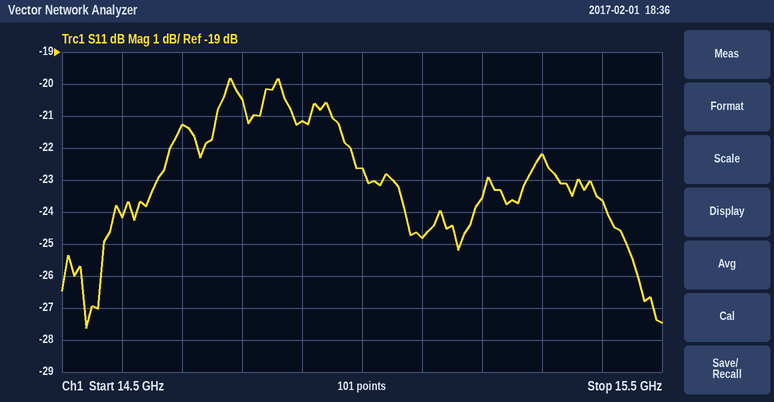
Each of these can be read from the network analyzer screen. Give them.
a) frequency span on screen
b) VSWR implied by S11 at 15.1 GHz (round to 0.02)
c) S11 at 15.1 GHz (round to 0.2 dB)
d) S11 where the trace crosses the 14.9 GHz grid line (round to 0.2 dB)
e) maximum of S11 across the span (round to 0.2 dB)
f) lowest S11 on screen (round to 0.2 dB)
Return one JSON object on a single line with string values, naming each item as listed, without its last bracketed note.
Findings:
{"frequency span on screen": "1 GHz", "VSWR implied by S11 at 15.1 GHz": "1.12", "S11 at 15.1 GHz": "-24.8 dB", "S11 where the trace crosses the 14.9 GHz grid line": "-21.2 dB", "maximum of S11 across the span": "-19.8 dB", "lowest S11 on screen": "-27.6 dB"}
